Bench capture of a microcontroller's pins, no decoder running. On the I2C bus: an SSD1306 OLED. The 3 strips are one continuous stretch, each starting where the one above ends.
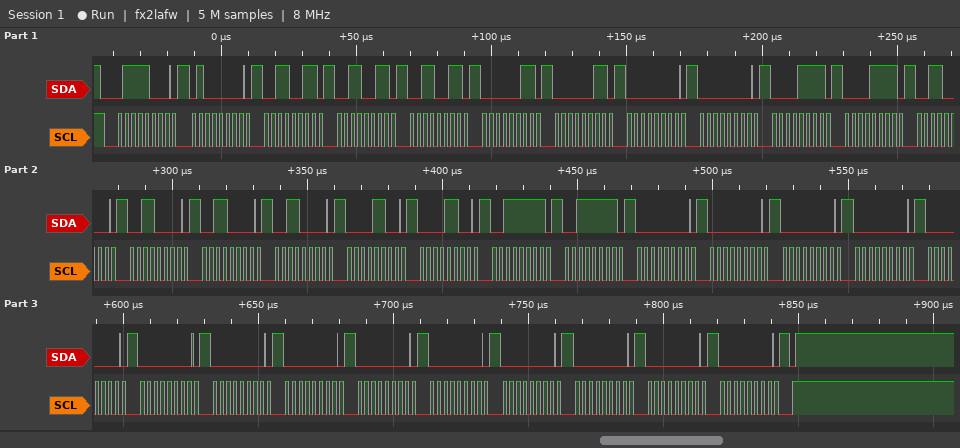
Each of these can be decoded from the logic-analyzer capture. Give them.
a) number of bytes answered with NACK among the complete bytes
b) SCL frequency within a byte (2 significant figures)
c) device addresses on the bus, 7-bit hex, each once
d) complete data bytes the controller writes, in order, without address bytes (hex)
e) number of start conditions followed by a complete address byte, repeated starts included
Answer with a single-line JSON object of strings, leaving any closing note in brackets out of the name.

{"number of bytes answered with NACK among the complete bytes": "0", "SCL frequency within a byte": "400 kHz", "device addresses on the bus, 7-bit hex, each once": "0x3C", "complete data bytes the controller writes, in order, without address bytes": "40 33 33 33 03 03 00 00 0F 0F 30 30 30 30 0C 0C 3F 3F 00 00 00 00 00 00 00 00 00 00 00 00 00 00", "number of start conditions followed by a complete address byte, repeated starts included": "1"}
